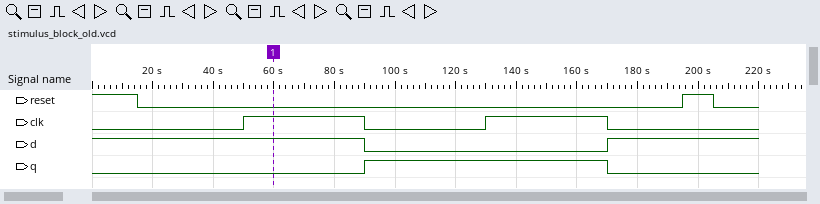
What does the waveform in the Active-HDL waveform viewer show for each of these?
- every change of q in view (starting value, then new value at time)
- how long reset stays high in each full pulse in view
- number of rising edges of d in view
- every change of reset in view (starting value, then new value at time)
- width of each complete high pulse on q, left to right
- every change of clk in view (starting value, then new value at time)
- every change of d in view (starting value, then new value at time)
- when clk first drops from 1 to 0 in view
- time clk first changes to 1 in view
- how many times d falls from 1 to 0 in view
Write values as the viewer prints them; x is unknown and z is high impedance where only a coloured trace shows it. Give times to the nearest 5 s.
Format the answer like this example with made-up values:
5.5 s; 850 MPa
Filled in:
0, 1 at 90 s, 0 at 170 s; 10 s; 1; 1, 0 at 15 s, 1 at 195 s, 0 at 205 s; 80 s; 0, 1 at 50 s, 0 at 90 s, 1 at 130 s, 0 at 170 s; 1, 0 at 90 s, 1 at 170 s; 90 s; 50 s; 1
